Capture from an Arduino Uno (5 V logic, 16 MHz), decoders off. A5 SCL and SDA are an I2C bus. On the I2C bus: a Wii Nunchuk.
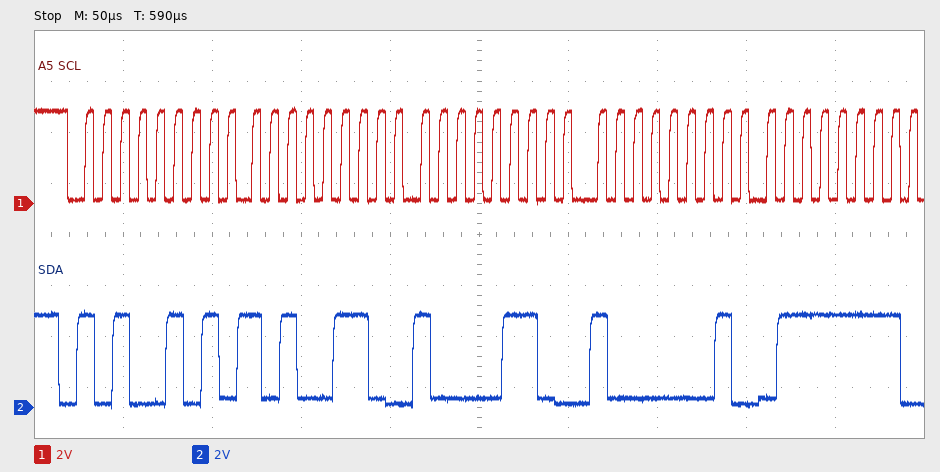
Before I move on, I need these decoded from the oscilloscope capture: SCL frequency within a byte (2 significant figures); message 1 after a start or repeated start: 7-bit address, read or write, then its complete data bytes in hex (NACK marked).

100 kHz
0x52 read: A6 86 81 7F
